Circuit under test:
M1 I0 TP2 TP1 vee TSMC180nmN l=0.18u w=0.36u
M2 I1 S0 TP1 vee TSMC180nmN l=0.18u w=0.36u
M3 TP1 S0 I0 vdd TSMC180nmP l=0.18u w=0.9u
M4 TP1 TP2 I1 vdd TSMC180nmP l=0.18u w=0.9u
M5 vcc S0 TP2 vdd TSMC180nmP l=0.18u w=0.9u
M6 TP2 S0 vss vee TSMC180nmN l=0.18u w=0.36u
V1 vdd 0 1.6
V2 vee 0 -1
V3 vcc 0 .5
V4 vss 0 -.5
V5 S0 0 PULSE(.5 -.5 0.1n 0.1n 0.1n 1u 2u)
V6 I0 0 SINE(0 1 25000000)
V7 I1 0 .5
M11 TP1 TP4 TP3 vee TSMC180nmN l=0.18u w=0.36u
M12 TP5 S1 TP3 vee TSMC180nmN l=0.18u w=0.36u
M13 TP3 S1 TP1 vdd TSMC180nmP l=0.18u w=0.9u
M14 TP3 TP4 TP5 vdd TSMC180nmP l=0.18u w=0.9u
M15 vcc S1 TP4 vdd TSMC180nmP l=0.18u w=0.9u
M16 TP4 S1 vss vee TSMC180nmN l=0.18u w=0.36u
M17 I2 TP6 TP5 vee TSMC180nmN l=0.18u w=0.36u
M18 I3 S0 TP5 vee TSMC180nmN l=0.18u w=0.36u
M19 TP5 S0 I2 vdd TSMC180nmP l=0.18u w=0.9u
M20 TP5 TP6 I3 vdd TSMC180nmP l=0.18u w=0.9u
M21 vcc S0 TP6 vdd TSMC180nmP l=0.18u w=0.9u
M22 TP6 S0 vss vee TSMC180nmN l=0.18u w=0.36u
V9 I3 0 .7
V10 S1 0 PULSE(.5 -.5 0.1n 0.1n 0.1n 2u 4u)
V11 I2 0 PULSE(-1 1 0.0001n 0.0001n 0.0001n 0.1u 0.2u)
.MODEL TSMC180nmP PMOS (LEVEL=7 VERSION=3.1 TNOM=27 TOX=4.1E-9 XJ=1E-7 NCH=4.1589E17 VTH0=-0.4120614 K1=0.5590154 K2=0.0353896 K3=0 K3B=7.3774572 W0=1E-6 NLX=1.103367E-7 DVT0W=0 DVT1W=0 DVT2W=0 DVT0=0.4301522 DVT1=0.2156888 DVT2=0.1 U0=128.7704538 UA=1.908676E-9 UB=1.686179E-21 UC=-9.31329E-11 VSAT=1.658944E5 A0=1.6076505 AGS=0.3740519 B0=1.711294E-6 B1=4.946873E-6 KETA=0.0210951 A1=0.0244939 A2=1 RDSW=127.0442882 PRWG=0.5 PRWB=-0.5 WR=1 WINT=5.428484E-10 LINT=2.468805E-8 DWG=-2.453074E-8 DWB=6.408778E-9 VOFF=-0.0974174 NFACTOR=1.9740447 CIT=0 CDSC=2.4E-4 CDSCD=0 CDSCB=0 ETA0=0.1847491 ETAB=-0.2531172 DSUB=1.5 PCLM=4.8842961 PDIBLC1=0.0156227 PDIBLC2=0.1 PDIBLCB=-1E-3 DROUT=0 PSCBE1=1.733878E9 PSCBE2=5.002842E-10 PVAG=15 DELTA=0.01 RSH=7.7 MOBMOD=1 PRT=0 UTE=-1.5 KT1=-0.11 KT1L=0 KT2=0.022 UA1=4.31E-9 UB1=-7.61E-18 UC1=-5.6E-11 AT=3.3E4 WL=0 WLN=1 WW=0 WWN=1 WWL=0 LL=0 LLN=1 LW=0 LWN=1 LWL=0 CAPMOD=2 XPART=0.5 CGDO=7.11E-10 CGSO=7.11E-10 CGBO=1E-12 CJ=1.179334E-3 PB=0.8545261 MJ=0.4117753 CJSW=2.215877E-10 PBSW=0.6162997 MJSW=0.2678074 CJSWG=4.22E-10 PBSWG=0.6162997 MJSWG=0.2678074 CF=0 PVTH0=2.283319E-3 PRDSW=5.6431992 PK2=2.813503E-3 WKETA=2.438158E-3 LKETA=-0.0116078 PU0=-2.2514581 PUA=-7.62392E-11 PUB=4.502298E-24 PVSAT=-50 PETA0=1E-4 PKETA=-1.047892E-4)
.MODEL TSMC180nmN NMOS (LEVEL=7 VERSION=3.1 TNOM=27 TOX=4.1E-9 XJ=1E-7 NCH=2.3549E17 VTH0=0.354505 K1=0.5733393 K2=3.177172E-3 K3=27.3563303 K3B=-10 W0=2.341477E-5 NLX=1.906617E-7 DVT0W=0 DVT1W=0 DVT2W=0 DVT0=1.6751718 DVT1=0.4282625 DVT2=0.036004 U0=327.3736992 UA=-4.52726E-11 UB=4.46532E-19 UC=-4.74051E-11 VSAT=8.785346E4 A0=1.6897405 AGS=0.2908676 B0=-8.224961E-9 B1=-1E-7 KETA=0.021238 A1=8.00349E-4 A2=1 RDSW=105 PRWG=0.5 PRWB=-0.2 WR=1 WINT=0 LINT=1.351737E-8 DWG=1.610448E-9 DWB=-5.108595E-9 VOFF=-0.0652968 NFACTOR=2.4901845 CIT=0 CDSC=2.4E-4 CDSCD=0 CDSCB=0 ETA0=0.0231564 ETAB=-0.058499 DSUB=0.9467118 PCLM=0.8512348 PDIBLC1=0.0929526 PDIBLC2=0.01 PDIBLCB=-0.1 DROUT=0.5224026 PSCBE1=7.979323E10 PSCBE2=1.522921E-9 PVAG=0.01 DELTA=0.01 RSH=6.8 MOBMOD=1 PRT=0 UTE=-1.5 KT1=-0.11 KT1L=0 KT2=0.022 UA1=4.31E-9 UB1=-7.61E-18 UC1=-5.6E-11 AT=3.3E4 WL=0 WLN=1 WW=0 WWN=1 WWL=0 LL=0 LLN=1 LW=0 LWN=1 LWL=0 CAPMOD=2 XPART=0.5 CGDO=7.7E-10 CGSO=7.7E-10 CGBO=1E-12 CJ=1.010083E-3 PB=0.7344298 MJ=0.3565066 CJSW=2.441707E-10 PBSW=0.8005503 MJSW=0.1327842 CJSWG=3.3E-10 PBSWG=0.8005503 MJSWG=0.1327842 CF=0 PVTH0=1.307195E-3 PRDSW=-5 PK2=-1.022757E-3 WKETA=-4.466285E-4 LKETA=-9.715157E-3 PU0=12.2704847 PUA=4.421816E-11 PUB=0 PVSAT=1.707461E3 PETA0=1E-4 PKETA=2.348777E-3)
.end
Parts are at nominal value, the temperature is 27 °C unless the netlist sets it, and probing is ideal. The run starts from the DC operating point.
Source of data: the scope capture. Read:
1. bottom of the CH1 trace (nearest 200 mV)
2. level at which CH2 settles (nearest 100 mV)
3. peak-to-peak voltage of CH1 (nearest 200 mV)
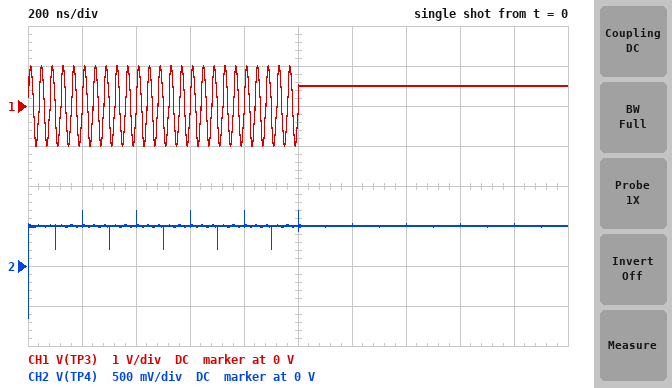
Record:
-1.0 V
500 mV
2.0 V
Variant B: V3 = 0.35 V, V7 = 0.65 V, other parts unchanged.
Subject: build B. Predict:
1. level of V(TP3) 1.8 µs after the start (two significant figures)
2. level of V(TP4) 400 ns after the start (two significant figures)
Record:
650 mV
350 mV
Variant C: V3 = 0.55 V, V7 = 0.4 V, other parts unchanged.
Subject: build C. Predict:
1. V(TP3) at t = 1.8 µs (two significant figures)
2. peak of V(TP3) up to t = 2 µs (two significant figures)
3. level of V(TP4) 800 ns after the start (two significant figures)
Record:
400 mV
1.0 V
550 mV
